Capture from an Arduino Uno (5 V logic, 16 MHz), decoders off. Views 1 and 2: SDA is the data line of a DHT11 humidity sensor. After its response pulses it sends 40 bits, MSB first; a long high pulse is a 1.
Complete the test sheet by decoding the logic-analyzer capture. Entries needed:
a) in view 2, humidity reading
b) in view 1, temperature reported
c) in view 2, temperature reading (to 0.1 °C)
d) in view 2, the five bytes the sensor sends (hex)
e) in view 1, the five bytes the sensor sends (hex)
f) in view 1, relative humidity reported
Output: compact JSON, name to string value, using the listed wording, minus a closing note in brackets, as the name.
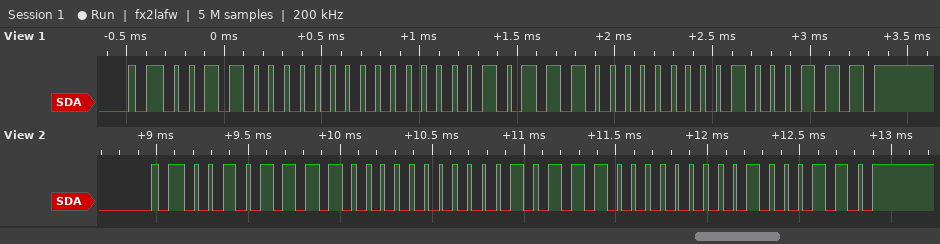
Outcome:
{"in view 2, humidity reading": "47 %", "in view 1, temperature reported": "23.0 °C", "in view 2, temperature reading": "23.0 °C", "in view 2, the five bytes the sensor sends": "2F 00 17 00 46", "in view 1, the five bytes the sensor sends": "30 00 17 00 47", "in view 1, relative humidity reported": "48 %"}
